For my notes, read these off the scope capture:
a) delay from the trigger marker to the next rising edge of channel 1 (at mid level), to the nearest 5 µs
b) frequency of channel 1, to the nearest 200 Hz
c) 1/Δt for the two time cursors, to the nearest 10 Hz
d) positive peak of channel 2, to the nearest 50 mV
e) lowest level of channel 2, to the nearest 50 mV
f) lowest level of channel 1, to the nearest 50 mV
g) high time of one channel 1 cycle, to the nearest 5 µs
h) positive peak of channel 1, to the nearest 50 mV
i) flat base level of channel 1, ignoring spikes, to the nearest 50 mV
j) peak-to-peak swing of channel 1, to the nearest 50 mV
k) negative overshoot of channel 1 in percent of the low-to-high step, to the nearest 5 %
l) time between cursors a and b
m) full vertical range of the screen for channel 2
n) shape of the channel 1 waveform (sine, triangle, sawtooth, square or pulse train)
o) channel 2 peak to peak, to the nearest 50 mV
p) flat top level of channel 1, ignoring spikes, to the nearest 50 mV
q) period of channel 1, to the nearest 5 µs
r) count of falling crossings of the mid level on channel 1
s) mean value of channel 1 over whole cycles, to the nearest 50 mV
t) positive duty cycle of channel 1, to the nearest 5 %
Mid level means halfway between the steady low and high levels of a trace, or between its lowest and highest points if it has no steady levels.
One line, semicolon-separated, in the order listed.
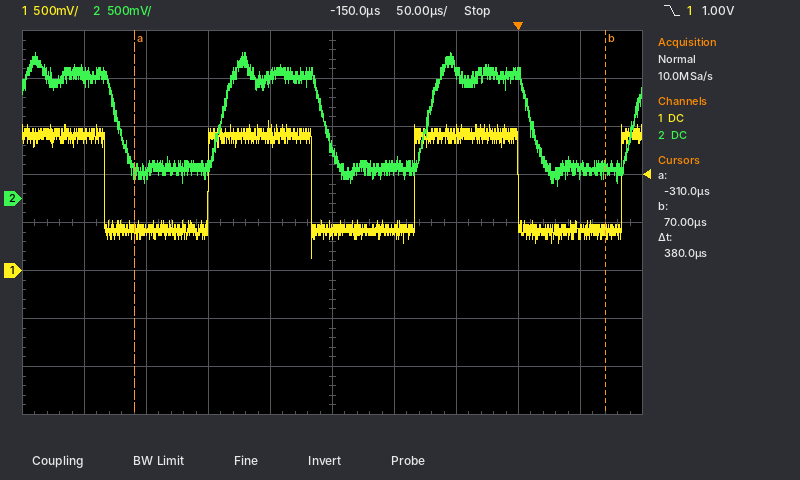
85 µs; 6.0 kHz; 2.63 kHz; 1.50 V; 100 mV; 100 mV; 85 µs; 1.55 V; 400 mV; 1.45 V; 30 %; 380 µs; 4 V; square; 1.40 V; 1.40 V; 165 µs; 3; 900 mV; 50 %
